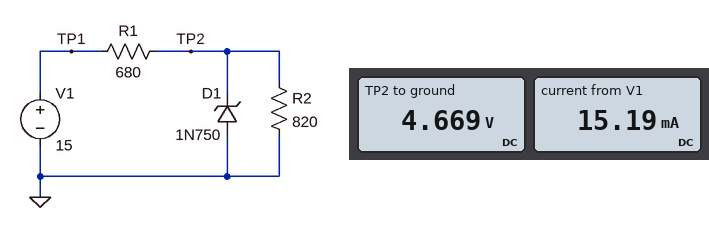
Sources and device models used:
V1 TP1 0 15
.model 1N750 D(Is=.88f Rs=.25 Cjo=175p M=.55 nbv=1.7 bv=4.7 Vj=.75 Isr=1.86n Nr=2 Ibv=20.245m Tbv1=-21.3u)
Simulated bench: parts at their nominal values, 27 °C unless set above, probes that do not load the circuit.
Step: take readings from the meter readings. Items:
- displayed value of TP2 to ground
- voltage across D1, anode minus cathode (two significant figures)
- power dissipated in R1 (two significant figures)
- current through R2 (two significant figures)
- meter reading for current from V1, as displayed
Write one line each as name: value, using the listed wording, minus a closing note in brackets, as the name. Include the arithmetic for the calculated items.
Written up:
displayed value of TP2 to ground: 4.669 V
voltage across D1, anode minus cathode: 0 V - 4.669 V = -4.7 V
power dissipated in R1: (15 V - 4.669 V)^2 / 680 Ω = 160 mW
current through R2: (4.669 V) / 820 Ω = 5.7 mA
meter reading for current from V1, as displayed: 15.19 mA
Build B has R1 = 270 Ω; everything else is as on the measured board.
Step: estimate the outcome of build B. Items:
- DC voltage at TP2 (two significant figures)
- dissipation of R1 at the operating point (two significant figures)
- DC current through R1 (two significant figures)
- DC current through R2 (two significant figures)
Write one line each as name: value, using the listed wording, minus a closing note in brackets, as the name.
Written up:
DC voltage at TP2: 4.7 V
dissipation of R1 at the operating point: 390 mW
DC current through R1: 38 mA
DC current through R2: 5.8 mA
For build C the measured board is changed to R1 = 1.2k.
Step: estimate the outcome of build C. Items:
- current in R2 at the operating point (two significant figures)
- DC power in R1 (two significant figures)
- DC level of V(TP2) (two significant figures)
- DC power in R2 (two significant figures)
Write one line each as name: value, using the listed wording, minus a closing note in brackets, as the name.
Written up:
current in R2 at the operating point: 5.6 mA
DC power in R1: 90 mW
DC level of V(TP2): 4.6 V
DC power in R2: 26 mW
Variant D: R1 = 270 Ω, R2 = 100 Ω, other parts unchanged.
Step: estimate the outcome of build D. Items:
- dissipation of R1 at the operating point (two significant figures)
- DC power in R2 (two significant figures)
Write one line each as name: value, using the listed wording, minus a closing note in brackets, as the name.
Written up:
dissipation of R1 at the operating point: 440 mW
DC power in R2: 160 mW
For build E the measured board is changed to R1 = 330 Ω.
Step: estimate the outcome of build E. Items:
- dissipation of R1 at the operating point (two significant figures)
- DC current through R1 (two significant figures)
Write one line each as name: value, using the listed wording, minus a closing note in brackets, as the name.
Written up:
dissipation of R1 at the operating point: 320 mW
DC current through R1: 31 mA
